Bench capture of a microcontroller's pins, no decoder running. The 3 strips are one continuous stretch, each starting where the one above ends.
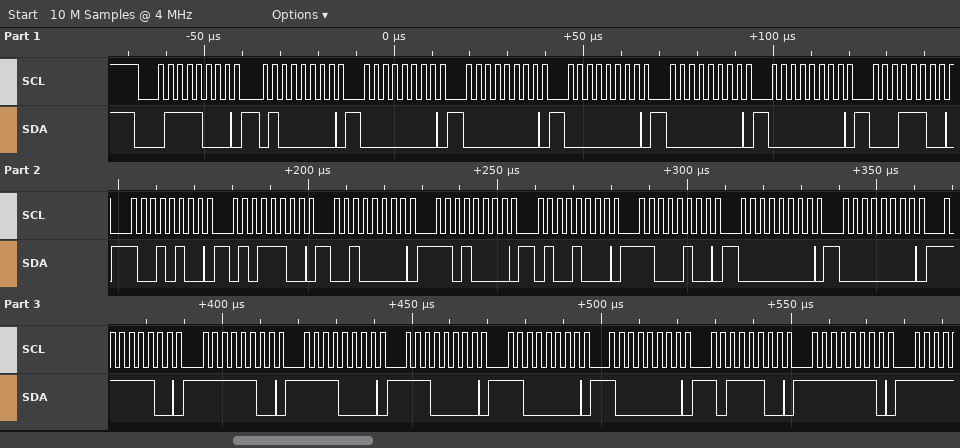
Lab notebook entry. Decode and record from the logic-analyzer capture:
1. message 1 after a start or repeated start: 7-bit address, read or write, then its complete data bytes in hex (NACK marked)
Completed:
0x3C write: 40 00 00 00 00 00 1C 94 5C 20 D0 48 C4 00 00 FC FC F0 E0 C0 80 BC FE
